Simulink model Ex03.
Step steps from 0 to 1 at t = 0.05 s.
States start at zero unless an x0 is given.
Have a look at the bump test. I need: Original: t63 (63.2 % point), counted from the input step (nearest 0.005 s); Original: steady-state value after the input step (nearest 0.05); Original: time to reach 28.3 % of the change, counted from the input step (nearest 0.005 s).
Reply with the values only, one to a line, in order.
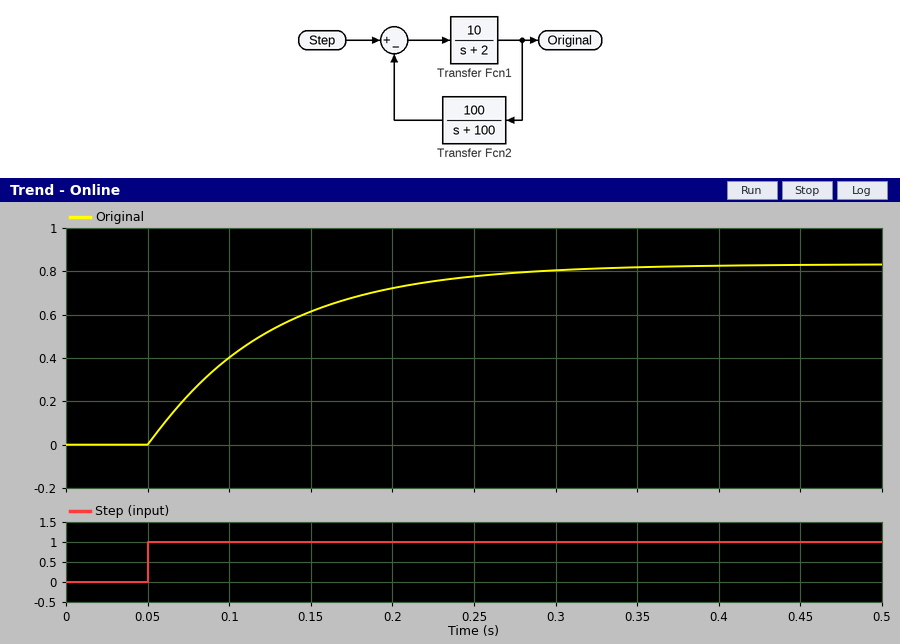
0.075 s
0.85
0.025 s
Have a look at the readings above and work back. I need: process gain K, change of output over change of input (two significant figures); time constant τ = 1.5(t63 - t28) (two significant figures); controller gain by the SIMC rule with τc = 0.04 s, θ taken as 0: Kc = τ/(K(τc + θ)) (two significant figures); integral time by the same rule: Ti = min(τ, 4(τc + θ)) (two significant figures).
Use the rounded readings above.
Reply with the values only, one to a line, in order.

0.85
0.075 s
2.2
0.075 s
